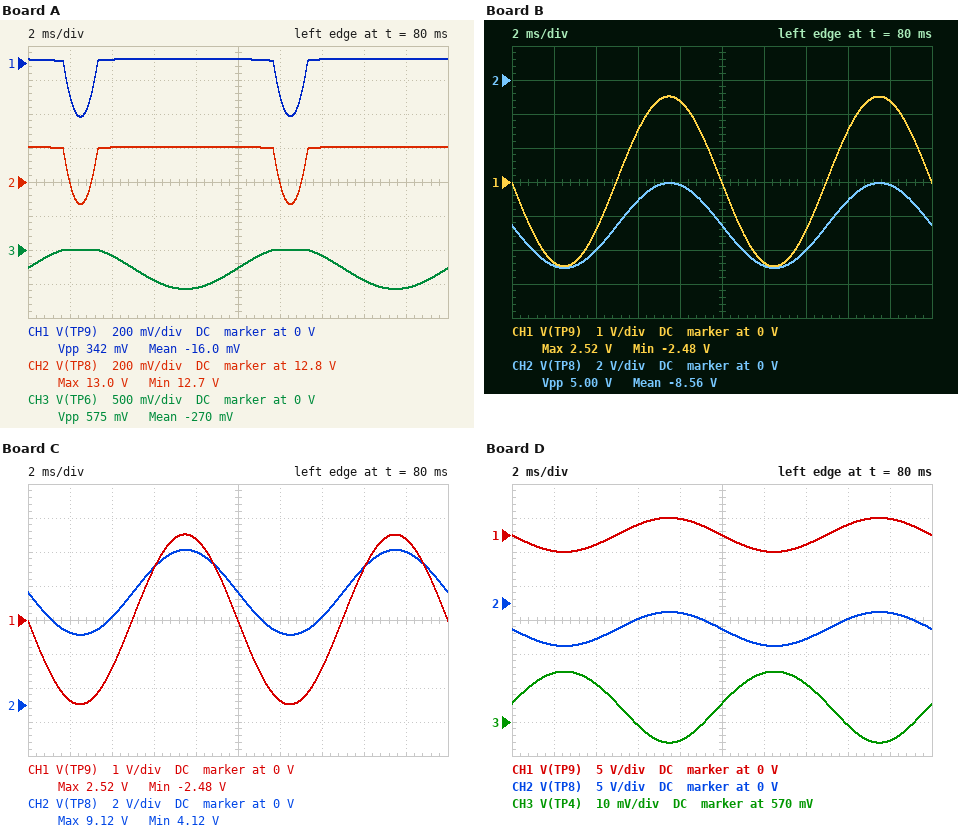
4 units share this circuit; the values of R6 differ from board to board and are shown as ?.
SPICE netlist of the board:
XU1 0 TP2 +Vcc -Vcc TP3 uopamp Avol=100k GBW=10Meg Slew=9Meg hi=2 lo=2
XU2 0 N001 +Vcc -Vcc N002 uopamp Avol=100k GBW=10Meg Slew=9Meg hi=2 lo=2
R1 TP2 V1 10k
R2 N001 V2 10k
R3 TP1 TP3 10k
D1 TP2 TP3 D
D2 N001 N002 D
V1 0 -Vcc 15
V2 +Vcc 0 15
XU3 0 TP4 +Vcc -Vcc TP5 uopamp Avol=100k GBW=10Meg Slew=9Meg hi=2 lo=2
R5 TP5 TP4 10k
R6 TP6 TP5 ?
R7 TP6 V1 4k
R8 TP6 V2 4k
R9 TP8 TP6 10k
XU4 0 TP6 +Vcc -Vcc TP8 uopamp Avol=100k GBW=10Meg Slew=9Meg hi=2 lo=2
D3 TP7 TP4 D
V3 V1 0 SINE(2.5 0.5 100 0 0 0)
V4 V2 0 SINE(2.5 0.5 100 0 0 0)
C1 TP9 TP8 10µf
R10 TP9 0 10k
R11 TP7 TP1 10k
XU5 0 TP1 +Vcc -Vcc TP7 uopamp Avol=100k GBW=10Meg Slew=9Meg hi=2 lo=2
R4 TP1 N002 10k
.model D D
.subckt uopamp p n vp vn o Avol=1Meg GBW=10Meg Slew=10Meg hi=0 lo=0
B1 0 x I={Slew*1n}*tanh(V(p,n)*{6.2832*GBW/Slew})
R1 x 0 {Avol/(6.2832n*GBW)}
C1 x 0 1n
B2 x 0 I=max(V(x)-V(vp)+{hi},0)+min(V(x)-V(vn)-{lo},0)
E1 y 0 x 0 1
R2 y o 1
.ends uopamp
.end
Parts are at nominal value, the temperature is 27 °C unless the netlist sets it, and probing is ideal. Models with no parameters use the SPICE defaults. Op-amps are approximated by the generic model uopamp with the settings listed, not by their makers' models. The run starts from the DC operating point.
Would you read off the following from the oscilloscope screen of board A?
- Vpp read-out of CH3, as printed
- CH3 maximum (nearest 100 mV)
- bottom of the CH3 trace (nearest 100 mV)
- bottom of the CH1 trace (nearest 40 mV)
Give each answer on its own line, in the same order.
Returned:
575 mV
0 V
-600 mV
-320 mV
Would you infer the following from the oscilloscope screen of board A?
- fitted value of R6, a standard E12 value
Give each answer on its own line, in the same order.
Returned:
4.7 kΩ
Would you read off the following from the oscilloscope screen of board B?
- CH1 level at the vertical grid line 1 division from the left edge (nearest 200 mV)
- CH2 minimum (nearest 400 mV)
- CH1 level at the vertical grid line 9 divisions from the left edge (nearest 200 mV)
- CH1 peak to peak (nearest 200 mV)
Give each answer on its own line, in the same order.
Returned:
-2.4 V
-11.2 V
2.4 V
5.0 V
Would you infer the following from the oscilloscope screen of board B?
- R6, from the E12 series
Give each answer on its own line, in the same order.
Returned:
33 kΩ
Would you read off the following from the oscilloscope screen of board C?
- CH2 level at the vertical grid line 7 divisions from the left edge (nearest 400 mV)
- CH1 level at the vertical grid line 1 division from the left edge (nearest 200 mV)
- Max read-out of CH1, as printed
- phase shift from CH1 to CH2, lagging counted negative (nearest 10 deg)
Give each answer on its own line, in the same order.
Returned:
5.2 V
-2.4 V
2.52 V
0 deg
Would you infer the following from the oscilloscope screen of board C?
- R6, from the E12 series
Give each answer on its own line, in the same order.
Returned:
6.8 kΩ
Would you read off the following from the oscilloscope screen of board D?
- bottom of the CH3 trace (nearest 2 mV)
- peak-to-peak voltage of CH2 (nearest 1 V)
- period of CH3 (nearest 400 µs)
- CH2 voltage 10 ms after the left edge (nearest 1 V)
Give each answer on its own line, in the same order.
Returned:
564 mV
5 V
10.0 ms
-4 V
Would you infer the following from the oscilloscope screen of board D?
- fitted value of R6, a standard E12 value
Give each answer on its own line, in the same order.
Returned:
15 kΩ
